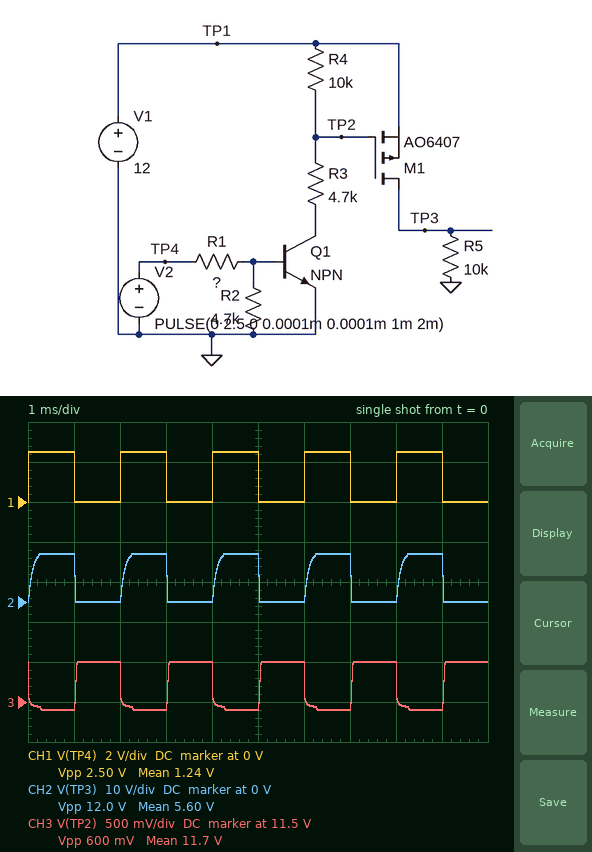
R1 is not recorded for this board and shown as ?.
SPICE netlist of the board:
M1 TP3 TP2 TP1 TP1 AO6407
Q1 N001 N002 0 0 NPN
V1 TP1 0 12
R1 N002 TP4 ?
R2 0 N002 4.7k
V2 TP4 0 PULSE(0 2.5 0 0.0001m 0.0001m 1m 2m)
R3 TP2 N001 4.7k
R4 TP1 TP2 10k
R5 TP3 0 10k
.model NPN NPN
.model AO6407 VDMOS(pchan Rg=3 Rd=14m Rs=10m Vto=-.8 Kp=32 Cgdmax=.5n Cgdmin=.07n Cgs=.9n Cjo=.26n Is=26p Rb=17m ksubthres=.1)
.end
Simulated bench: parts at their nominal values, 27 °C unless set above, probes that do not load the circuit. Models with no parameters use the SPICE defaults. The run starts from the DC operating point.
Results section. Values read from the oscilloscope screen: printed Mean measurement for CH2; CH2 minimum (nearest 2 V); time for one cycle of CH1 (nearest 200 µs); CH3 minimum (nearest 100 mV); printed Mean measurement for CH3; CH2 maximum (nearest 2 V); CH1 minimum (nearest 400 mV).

5.60 V
0 V
2.0 ms
11.4 V
11.7 V
12 V
0 V
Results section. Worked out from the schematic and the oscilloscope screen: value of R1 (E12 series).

12 kΩ
